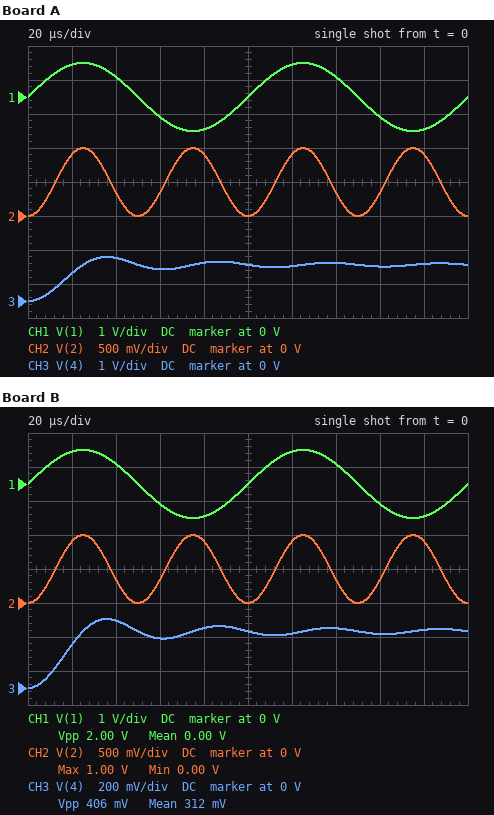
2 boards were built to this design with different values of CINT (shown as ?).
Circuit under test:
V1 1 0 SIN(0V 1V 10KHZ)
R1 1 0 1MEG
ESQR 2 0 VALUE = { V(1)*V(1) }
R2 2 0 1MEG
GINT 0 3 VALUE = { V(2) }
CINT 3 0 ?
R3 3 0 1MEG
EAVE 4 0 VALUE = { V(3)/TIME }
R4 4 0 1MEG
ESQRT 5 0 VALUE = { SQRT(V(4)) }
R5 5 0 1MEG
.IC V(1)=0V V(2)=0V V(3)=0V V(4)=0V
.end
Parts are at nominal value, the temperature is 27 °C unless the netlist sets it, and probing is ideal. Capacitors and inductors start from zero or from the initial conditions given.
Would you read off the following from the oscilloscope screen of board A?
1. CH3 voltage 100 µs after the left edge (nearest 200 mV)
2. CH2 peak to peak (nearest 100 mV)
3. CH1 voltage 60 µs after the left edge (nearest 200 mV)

1.0 V
1.0 V
-600 mV
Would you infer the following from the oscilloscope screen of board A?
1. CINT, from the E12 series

470 mF
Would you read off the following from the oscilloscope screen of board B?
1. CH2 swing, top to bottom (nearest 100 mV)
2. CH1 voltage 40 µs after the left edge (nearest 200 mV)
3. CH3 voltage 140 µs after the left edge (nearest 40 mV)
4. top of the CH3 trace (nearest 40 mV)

1.0 V
600 mV
360 mV
400 mV
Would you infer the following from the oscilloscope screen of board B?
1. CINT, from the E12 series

1.5 F
